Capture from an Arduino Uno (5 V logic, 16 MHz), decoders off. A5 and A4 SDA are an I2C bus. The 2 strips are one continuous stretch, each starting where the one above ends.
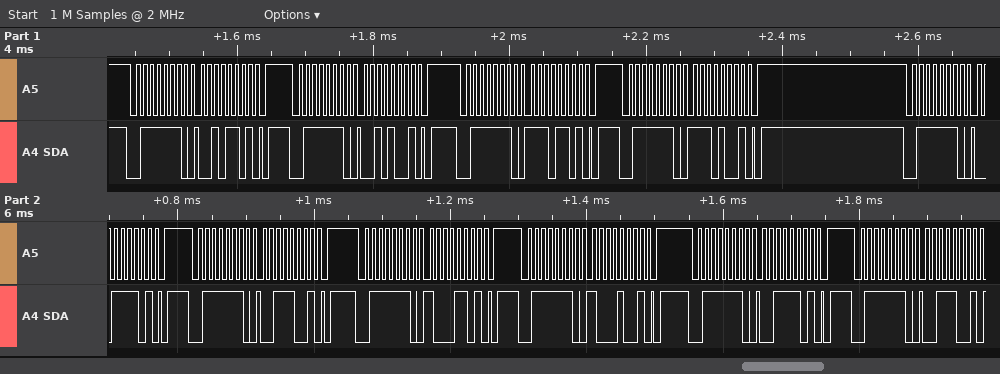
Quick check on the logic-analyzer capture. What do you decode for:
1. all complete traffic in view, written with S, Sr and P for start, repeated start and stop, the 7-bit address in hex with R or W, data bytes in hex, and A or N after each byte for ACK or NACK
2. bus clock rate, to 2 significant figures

S 3FW A 2D A P S 3FW A 29 A P S 3FW A ED A P S 3FW A E9 A P S 3FW A 3D A P S 3FW A 39 A P S 3FW A 8D A P S 3FW A 89 A P S 3FW A 3D A P S 3FW A 39 A
100 kHz
